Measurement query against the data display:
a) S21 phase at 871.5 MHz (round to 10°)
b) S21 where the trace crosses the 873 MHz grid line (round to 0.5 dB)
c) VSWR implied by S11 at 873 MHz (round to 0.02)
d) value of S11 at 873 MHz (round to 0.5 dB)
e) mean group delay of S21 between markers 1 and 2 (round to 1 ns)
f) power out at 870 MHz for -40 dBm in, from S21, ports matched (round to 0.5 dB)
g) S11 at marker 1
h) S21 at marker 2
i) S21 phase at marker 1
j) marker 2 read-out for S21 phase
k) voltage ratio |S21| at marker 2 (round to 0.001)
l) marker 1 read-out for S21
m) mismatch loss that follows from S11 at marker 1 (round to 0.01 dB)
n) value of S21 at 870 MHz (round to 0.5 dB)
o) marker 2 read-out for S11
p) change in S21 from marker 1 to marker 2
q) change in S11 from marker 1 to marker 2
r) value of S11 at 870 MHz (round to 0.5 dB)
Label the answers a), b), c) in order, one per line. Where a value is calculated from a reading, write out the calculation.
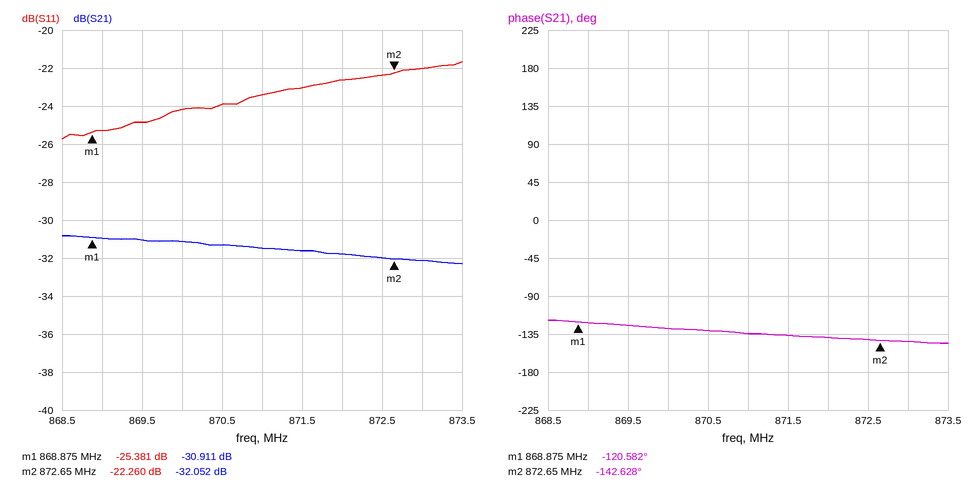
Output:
a) -140°
b) -32.0 dB
c) |Γ| = 10^(-22/20) = 0.0794; VSWR = (1 + 0.0794)/(1 − 0.0794) ≈ 1.17, so 1.18 to the nearest 0.02
d) -22.0 dB
e) −(-142.628° − (-120.582°))/(360° × 3.775 MHz) ≈ 16 ns
f) -40 dBm + (-31.0 dB) = -71.0 dBm
g) -25.381 dB
h) -32.052 dB
i) -120.582°
j) -142.628°
k) 10^(-32.052/20) ≈ 0.025
l) -30.911 dB
m) −10 log10(1 − 10^(-25.381/10)) ≈ 0.01 dB
n) -31.0 dB
o) -22.260 dB
p) -32.052 − (-30.911) = -1.141 dB
q) -22.26 − (-25.381) = 3.121 dB
r) -24.0 dB
